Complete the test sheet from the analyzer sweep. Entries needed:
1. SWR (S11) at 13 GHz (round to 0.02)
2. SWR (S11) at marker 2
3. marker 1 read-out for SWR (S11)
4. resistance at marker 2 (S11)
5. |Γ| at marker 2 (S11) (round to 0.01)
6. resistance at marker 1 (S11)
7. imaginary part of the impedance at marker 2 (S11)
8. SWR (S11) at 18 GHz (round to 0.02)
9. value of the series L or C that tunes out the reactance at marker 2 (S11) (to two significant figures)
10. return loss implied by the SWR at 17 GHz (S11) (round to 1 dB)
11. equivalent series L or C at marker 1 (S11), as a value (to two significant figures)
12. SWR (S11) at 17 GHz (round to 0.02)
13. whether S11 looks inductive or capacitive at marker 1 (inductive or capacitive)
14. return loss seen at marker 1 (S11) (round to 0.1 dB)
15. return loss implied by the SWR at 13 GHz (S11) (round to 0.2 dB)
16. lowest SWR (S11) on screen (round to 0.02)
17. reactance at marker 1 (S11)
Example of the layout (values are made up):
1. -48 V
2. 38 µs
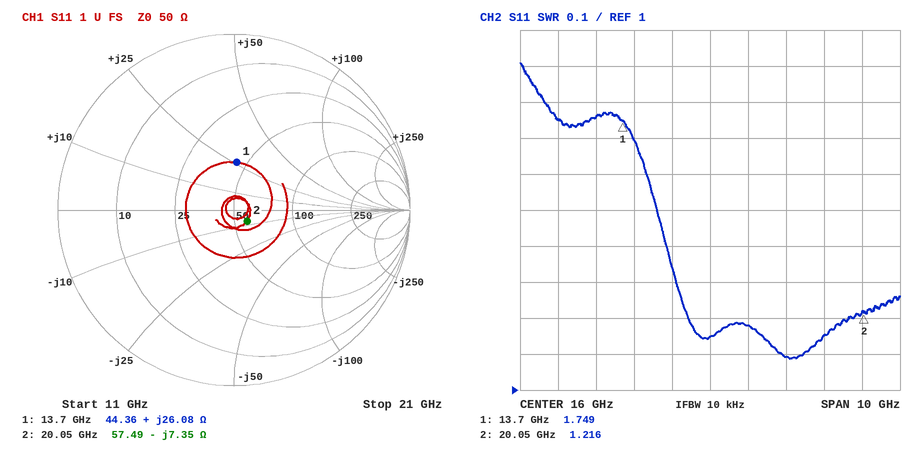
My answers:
1. 1.76
2. 1.216
3. 1.749
4. 57.49 Ω
5. 0.10
6. 44.36 Ω
7. -7.35 Ω
8. 1.10
9. 58 pH
10. 22 dB
11. 300 pH
12. 1.18
13. inductive
14. 11.3 dB
15. 11.2 dB
16. 1.08
17. +26.08 Ω
